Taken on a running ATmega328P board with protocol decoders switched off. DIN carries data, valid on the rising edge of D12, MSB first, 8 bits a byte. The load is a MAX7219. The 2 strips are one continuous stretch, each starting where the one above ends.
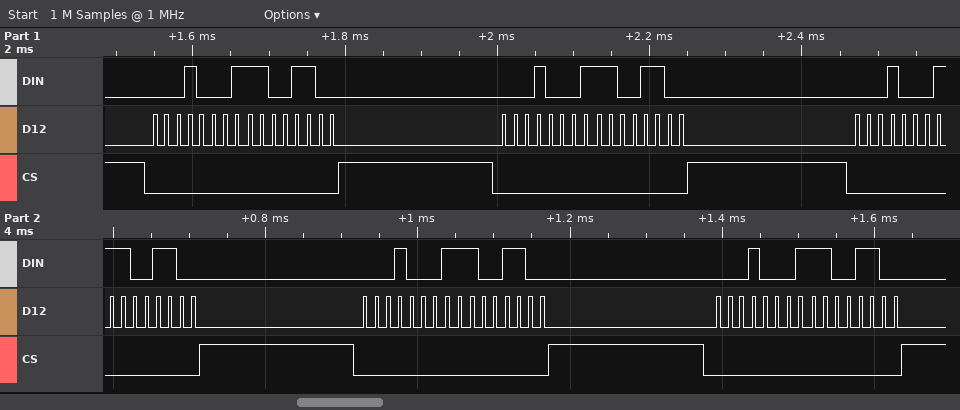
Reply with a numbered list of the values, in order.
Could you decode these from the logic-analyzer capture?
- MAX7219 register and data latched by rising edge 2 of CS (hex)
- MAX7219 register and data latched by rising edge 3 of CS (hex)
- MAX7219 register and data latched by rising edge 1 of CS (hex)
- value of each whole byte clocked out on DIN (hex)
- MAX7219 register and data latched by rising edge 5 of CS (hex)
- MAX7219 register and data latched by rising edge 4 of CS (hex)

1. register 0x1, data 0xCC
2. register 0x1, data 0xCC
3. register 0x1, data 0xCC
4. 0x11 0xCC 0x11 0xCC 0x11 0xCC 0x11 0xCC 0x11 0xCC
5. register 0x1, data 0xCC
6. register 0x1, data 0xCC
